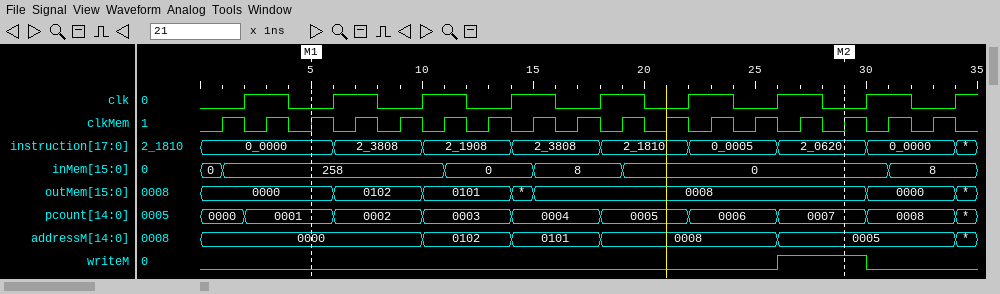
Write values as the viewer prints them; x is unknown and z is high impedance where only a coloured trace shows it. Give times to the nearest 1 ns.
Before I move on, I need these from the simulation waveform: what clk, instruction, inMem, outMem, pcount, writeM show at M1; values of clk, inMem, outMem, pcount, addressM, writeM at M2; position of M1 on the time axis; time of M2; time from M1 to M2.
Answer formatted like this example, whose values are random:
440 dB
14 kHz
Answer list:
clk=0, instruction=0_0000, inMem=258, outMem=0000, pcount=0001, writeM=0
clk=0, inMem=0, outMem=0008, pcount=0007, addressM=0005, writeM=1
5 ns
29 ns
24 ns
